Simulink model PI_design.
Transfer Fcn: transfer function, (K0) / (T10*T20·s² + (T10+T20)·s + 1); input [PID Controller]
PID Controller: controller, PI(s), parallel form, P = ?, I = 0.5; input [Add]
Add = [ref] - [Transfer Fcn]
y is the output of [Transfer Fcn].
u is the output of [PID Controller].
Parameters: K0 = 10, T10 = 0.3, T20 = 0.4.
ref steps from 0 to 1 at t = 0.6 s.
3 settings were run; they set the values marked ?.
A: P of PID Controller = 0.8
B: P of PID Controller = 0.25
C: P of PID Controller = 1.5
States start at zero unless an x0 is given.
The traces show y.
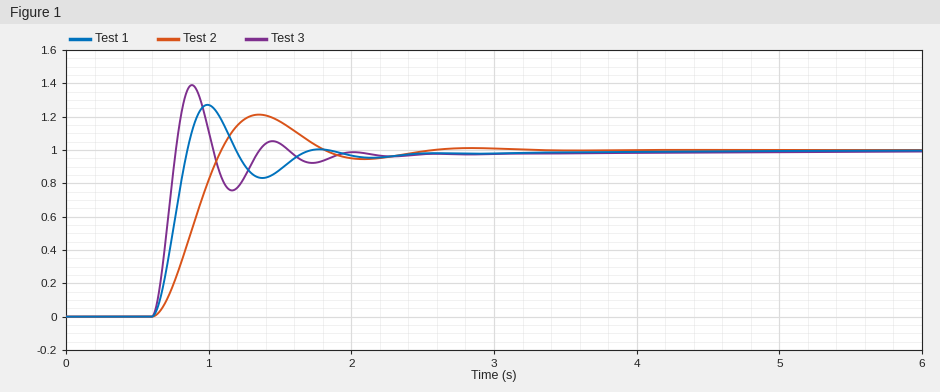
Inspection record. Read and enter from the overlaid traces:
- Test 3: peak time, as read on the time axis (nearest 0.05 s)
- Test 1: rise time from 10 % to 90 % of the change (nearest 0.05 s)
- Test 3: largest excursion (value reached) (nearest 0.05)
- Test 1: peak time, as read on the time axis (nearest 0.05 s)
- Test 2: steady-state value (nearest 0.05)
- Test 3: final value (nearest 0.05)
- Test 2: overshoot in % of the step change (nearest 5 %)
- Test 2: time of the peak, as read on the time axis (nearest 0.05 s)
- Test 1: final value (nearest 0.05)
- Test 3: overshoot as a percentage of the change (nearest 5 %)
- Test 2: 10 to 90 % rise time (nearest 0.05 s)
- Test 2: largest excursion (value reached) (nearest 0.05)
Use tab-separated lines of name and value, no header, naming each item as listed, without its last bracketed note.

Test 3: peak time, as read on the time axis	0.90 s
Test 1: rise time from 10 % to 90 % of the change	0.15 s
Test 3: largest excursion (value reached)	1.40
Test 1: peak time, as read on the time axis	1.00 s
Test 2: steady-state value	1.00
Test 3: final value	1.00
Test 2: overshoot in % of the step change	20 %
Test 2: time of the peak, as read on the time axis	1.35 s
Test 1: final value	1.00
Test 3: overshoot as a percentage of the change	40 %
Test 2: 10 to 90 % rise time	0.35 s
Test 2: largest excursion (value reached)	1.20
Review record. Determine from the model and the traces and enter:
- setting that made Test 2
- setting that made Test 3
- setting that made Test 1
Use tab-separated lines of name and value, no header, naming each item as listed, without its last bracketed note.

setting that made Test 2	B
setting that made Test 3	C
setting that made Test 1	A
